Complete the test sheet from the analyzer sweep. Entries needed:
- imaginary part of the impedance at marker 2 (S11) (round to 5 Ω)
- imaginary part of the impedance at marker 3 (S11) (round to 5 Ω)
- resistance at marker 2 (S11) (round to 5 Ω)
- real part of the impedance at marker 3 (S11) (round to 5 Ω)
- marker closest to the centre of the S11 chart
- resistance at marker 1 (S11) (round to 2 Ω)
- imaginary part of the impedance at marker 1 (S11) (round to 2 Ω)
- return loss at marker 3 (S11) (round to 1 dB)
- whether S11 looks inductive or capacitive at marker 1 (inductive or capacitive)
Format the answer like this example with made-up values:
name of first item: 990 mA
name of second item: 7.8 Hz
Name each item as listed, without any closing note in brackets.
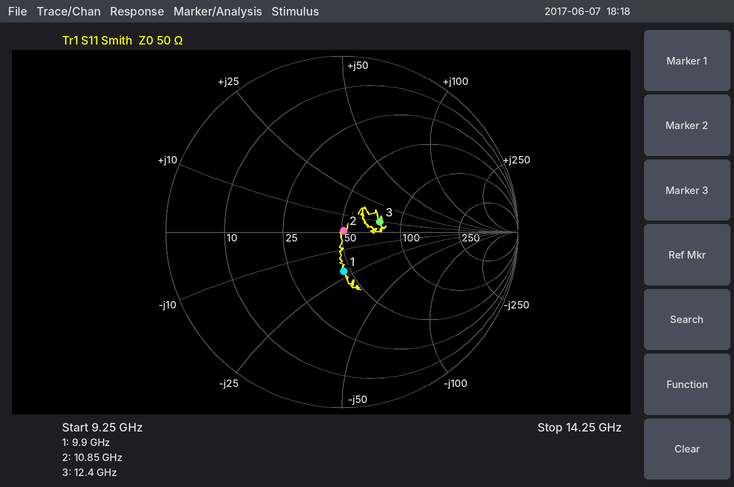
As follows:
imaginary part of the impedance at marker 2 (S11): 0 Ω
imaginary part of the impedance at marker 3 (S11): +10 Ω
resistance at marker 2 (S11): 50 Ω
real part of the impedance at marker 3 (S11): 75 Ω
marker closest to the centre of the S11 chart: marker 2
resistance at marker 1 (S11): 46 Ω
imaginary part of the impedance at marker 1 (S11): -22 Ω
return loss at marker 3 (S11): 13 dB
whether S11 looks inductive or capacitive at marker 1: capacitive
